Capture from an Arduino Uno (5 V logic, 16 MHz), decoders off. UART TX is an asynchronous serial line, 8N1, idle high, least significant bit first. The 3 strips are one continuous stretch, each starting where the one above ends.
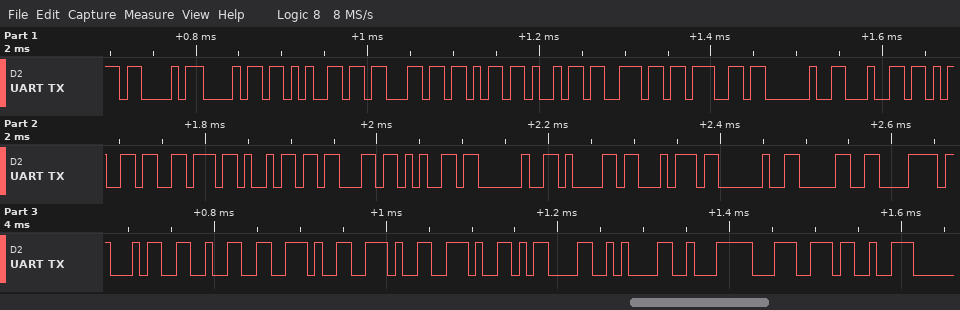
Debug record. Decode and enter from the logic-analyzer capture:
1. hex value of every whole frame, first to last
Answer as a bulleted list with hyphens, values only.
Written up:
- 0x43 0x68 0x65 0x63 0x6B 0x69 0x6E 0x67 0x20 0x64 0x65 0x76 0x69 0x63 0x65 0x20 0x61 0x74 0x20 0x30 0x78 0x34 0x32 0x2E 0x2E 0x2E 0x0D 0x0A 0xE2 0x9C 0x93
